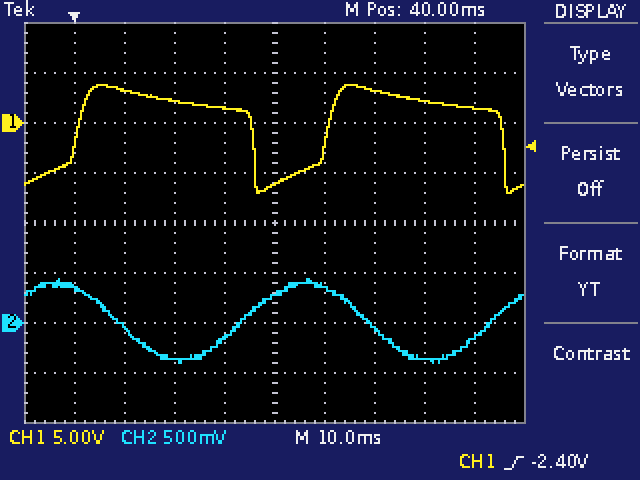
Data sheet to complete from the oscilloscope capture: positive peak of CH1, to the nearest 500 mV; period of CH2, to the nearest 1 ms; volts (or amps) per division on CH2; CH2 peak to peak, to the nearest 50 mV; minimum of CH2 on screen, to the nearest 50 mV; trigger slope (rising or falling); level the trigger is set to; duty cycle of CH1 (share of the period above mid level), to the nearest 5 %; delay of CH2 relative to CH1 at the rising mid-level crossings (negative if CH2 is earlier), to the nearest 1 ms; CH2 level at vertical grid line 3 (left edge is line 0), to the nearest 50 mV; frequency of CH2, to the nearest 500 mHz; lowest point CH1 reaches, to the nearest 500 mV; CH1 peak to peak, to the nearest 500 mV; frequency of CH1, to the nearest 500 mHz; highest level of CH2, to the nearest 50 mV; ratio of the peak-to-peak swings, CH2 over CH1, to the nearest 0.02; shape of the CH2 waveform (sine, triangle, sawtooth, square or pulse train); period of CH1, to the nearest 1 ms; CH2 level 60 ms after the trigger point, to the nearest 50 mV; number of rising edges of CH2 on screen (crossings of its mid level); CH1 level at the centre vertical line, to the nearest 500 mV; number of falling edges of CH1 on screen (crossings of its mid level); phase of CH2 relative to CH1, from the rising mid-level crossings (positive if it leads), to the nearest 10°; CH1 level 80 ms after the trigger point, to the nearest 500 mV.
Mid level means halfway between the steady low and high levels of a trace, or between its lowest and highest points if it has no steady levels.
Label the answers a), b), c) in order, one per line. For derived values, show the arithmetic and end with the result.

a) 4.0 V
b) 50 ms
c) 500 mV
d) 450 mV − (-400 mV) = 850 mV
e) -400 mV
f) rising
g) -2.40 V
h) 70 %
i) -17 ms
j) -350 mV
k) 1 / 50 ms ≈ 20.0 Hz
l) -7.0 V
m) 4.0 V − (-7.0 V) = 11.0 V
n) 1 / 50 ms ≈ 20.0 Hz
o) 450 mV
p) 850 mV / 11.0 V ≈ 0.08
q) sine
r) 50 ms
s) -50 mV
t) 2
u) -6.0 V
v) 2
w) −360° × (-17 ms) / 50 ms ≈ +122°, so +120° to the nearest 10°
x) 1.5 V
